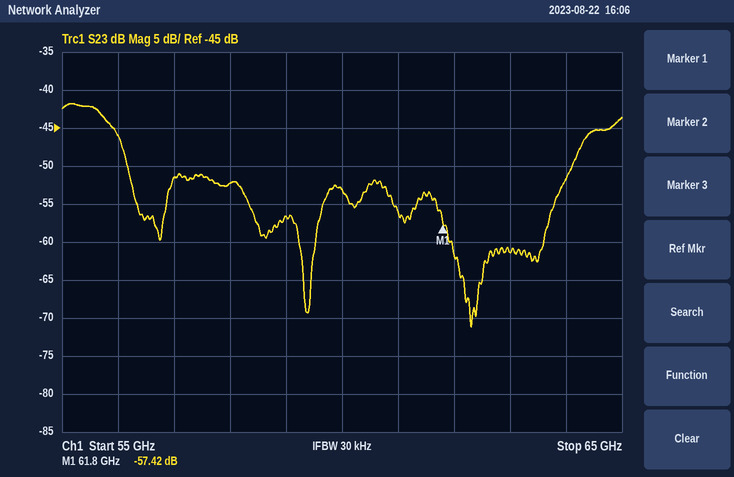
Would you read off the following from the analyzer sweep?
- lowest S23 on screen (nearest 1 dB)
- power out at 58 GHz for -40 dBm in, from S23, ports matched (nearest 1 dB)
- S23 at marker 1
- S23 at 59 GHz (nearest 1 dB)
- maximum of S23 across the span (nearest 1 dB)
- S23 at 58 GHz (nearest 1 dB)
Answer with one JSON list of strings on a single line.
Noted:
["-71 dB", "-92 dBm", "-57.42 dB", "-57 dB", "-42 dB", "-52 dB"]
